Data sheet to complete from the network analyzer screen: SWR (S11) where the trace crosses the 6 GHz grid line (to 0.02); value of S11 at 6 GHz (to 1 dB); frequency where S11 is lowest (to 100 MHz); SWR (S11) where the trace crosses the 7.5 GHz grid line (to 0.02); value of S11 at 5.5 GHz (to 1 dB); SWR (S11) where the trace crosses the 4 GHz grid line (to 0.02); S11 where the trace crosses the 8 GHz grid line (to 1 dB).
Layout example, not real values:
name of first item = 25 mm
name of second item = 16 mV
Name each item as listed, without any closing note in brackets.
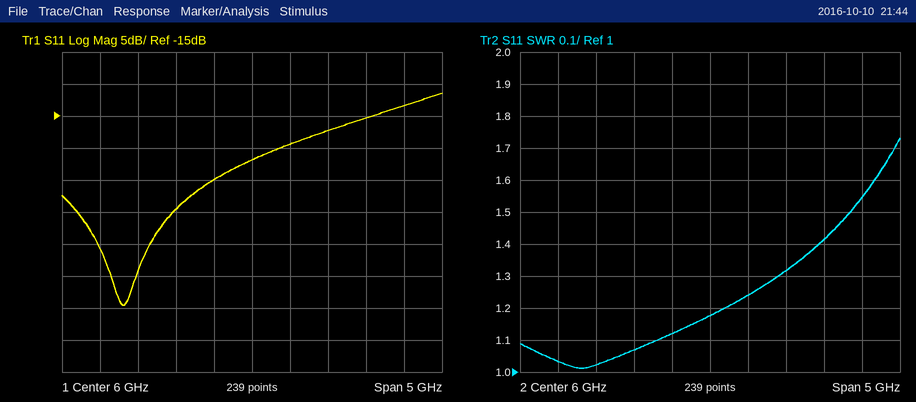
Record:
SWR (S11) where the trace crosses the 6 GHz grid line = 1.18
value of S11 at 6 GHz = -22 dB
frequency where S11 is lowest = 4.3 GHz
SWR (S11) where the trace crosses the 7.5 GHz grid line = 1.42
value of S11 at 5.5 GHz = -25 dB
SWR (S11) where the trace crosses the 4 GHz grid line = 1.04
S11 where the trace crosses the 8 GHz grid line = -13 dB
